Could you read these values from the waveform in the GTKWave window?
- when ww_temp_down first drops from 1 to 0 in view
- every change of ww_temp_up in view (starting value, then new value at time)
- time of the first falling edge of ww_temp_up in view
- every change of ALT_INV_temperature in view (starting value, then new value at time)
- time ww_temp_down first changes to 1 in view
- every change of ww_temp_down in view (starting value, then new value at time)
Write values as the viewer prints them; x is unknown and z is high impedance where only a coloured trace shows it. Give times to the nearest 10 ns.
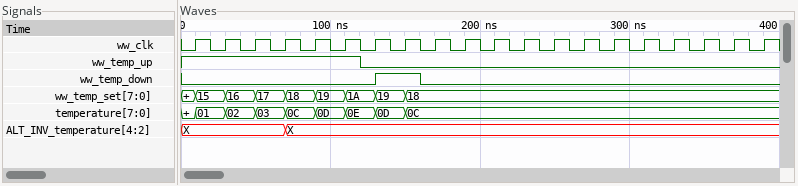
160 ns
1, 0 at 120 ns
120 ns
X, X at 70 ns
130 ns
0, 1 at 130 ns, 0 at 160 ns
